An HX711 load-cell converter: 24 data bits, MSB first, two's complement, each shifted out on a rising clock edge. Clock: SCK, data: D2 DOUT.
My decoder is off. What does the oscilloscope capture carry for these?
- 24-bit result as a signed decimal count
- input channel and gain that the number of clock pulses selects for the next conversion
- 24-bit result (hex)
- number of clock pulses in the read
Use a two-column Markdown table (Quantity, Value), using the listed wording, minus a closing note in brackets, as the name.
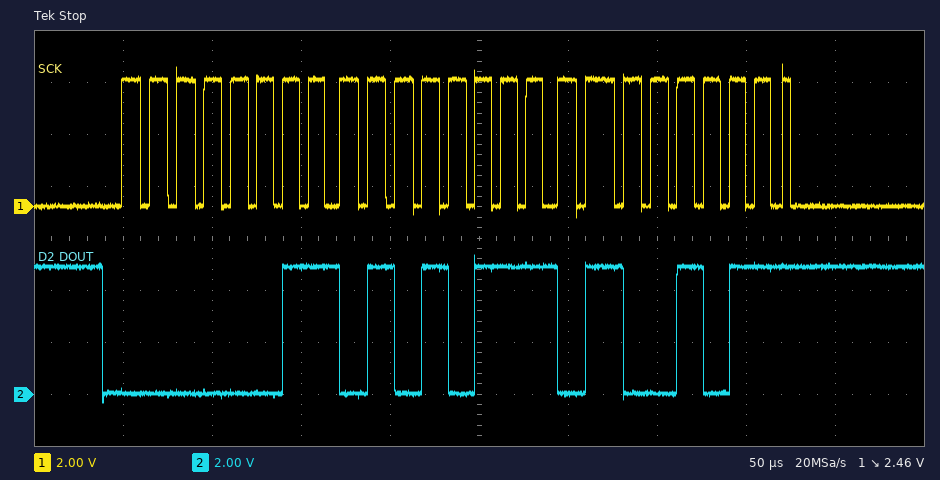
| Quantity | Value |
|---|---|
| 24-bit result as a signed decimal count | 218955 |
| input channel and gain that the number of clock pulses selects for the next conversion | channel A, gain 128 |
| 24-bit result | 0x03574B |
| number of clock pulses in the read | 25 |
